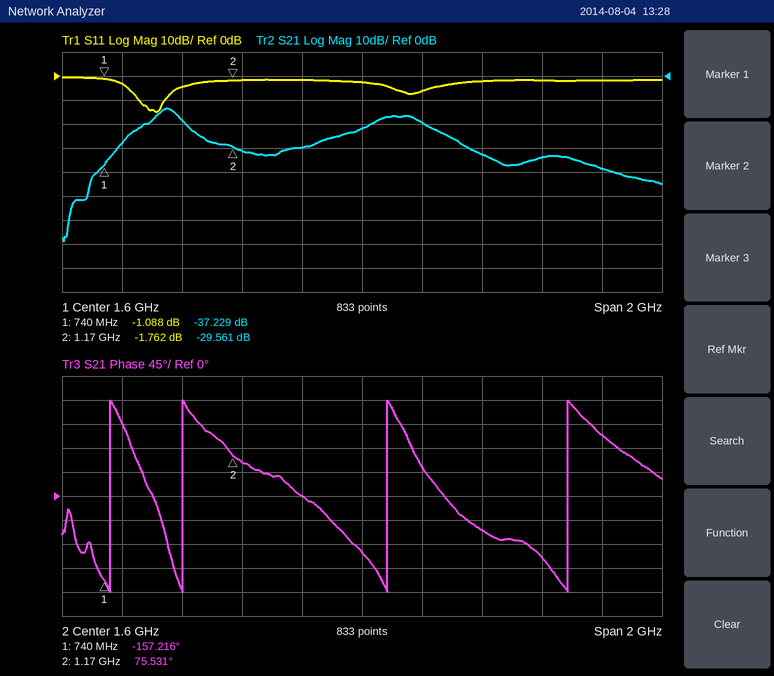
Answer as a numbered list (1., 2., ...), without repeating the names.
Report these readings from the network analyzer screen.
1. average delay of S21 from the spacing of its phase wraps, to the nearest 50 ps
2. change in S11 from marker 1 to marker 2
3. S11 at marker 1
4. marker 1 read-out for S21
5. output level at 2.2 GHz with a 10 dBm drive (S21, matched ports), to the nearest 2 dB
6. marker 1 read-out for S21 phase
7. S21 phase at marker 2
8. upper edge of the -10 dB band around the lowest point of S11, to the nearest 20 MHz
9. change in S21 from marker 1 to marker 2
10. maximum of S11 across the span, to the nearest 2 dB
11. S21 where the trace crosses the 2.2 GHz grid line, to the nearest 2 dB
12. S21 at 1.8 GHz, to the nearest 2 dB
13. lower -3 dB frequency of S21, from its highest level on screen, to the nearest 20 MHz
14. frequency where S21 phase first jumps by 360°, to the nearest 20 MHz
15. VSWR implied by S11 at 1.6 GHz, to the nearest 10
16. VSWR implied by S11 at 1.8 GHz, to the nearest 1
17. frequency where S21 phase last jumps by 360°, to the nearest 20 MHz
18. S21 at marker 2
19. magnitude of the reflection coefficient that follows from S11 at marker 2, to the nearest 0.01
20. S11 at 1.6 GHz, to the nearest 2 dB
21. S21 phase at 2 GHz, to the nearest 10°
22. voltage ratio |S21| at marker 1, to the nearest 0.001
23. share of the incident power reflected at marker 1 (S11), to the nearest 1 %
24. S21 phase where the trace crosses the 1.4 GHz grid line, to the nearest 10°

1. 1.95 ns
2. -0.674 dB
3. -1.088 dB
4. -37.229 dB
5. -24 dBm
6. -157.216°
7. 75.531°
8. 940 MHz
9. 7.668 dB
10. 0 dB
11. -34 dB
12. -20 dB
13. 920 MHz
14. 760 MHz
15. 10
16. 3
17. 2.28 GHz
18. -29.561 dB
19. 0.82
20. -2 dB
21. -60°
22. 0.014
23. 78 %
24. 0°
